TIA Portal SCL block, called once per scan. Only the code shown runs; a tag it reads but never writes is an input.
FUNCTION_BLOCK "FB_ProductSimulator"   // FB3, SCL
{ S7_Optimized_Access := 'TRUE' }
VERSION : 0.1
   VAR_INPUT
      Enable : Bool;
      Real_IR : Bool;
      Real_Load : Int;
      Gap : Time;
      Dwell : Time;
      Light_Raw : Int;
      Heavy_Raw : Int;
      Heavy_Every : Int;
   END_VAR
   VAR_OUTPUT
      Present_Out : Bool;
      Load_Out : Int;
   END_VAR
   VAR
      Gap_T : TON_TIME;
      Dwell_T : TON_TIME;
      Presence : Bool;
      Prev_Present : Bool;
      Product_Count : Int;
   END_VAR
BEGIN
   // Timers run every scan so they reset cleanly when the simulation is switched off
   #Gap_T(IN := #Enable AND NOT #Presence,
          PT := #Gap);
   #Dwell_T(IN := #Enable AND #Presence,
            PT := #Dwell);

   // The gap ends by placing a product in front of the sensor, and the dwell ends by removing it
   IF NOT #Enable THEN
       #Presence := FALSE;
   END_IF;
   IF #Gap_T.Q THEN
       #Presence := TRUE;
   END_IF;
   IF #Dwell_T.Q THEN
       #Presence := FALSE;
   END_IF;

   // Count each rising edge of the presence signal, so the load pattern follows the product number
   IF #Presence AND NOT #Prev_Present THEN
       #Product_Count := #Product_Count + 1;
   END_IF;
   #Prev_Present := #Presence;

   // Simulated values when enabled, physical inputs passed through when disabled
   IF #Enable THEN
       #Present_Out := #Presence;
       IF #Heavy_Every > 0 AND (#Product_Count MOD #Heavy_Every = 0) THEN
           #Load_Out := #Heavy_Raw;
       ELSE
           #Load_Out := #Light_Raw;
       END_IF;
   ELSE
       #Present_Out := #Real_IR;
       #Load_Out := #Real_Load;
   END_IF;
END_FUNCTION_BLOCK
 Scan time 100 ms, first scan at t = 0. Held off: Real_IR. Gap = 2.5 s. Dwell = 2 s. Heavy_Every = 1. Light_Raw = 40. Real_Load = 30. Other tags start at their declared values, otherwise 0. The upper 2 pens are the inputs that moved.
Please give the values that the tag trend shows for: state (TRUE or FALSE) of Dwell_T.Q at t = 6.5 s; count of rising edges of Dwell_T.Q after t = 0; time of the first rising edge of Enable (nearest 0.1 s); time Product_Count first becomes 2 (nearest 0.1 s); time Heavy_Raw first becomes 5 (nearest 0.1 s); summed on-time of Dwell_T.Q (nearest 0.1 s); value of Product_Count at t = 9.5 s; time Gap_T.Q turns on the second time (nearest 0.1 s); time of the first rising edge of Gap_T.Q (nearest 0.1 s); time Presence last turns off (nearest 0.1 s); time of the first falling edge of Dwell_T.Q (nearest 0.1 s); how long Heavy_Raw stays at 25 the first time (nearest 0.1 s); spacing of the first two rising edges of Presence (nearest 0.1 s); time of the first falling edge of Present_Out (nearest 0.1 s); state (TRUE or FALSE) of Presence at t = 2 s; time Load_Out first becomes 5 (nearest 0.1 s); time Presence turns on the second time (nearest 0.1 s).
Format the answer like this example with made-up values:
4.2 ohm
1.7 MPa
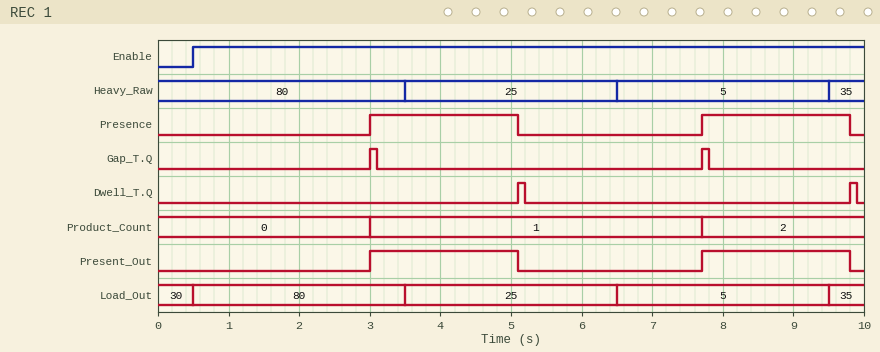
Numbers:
FALSE
2
0.5 s
7.7 s
6.5 s
0.2 s
2
7.7 s
3.0 s
9.8 s
5.2 s
3.0 s
4.7 s
5.1 s
FALSE
6.5 s
7.7 s
